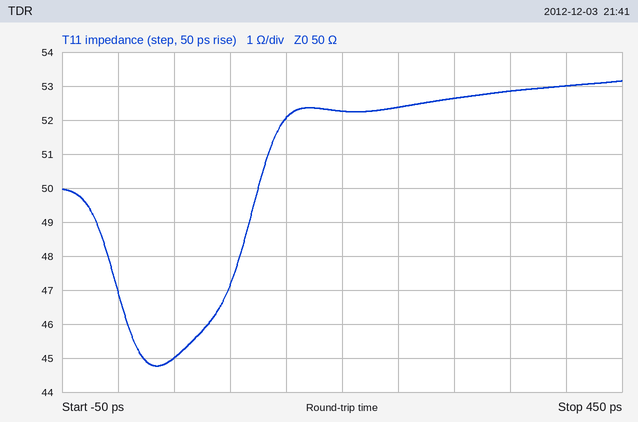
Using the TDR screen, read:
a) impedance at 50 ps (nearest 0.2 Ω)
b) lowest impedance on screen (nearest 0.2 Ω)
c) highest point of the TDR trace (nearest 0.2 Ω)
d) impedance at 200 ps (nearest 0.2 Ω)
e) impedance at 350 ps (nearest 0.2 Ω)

45.0 Ω
44.8 Ω
53.2 Ω
52.2 Ω
52.8 Ω
